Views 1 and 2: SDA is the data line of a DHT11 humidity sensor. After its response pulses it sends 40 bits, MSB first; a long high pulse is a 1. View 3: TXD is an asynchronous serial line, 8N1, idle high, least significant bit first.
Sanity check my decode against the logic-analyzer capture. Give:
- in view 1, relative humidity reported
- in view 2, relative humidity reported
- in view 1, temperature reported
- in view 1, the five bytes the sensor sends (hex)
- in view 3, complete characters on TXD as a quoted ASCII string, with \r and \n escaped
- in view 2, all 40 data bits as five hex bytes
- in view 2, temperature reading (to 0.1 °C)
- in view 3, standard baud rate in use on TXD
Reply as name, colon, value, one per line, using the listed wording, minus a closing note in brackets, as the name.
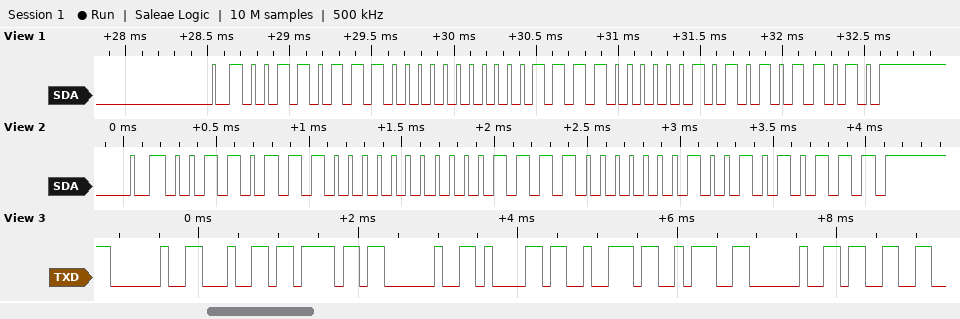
in view 1, relative humidity reported: 55 %
in view 2, relative humidity reported: 55 %
in view 1, temperature reported: 30.5 °C
in view 1, the five bytes the sensor sends: 37 00 1E 05 5A
in view 3, complete characters on TXD as a quoted ASCII string, with \r and \n escaped: " do ar: 3"
in view 2, all 40 data bits as five hex bytes: 37 00 1E 02 57
in view 2, temperature reading: 30.2 °C
in view 3, standard baud rate in use on TXD: 9600 baud
